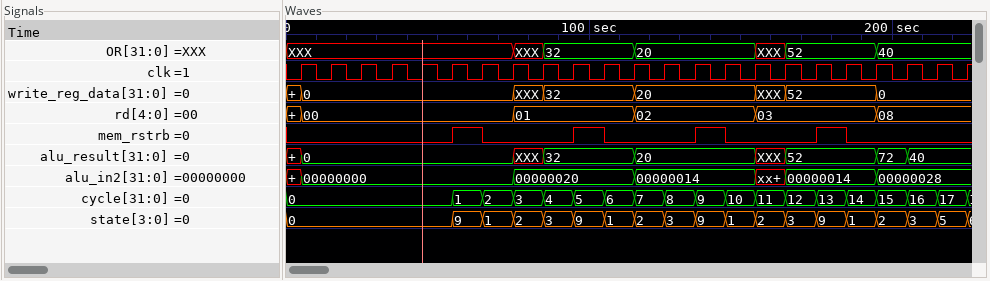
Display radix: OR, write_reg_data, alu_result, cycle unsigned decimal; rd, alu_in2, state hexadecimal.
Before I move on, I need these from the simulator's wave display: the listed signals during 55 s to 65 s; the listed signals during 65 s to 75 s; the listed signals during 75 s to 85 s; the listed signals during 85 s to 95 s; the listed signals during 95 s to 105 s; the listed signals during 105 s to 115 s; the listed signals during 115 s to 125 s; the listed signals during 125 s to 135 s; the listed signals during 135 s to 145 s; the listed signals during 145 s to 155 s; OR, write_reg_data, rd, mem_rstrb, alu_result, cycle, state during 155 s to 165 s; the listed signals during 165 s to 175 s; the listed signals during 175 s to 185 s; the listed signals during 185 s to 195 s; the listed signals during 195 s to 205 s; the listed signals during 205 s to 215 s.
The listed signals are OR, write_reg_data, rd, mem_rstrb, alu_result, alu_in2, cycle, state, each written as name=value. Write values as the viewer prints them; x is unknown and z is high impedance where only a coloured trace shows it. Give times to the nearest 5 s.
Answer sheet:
OR=XXX, write_reg_data=0, rd=00, mem_rstrb=1, alu_result=0, alu_in2=00000000, cycle=1, state=9
OR=XXX, write_reg_data=0, rd=00, mem_rstrb=0, alu_result=0, alu_in2=00000000, cycle=2, state=1
OR=XXX, write_reg_data=XXX, rd=01, mem_rstrb=0, alu_result=XXX, alu_in2=00000020, cycle=3, state=2
OR=32, write_reg_data=32, rd=01, mem_rstrb=0, alu_result=32, alu_in2=00000020, cycle=4, state=3
OR=32, write_reg_data=32, rd=01, mem_rstrb=1, alu_result=32, alu_in2=00000020, cycle=5, state=9
OR=32, write_reg_data=32, rd=01, mem_rstrb=0, alu_result=32, alu_in2=00000020, cycle=6, state=1
OR=20, write_reg_data=20, rd=02, mem_rstrb=0, alu_result=20, alu_in2=00000014, cycle=7, state=2
OR=20, write_reg_data=20, rd=02, mem_rstrb=0, alu_result=20, alu_in2=00000014, cycle=8, state=3
OR=20, write_reg_data=20, rd=02, mem_rstrb=1, alu_result=20, alu_in2=00000014, cycle=9, state=9
OR=20, write_reg_data=20, rd=02, mem_rstrb=0, alu_result=20, alu_in2=00000014, cycle=10, state=1
OR=XXX, write_reg_data=XXX, rd=03, mem_rstrb=0, alu_result=XXX, cycle=11, state=2
OR=52, write_reg_data=52, rd=03, mem_rstrb=0, alu_result=52, alu_in2=00000014, cycle=12, state=3
OR=52, write_reg_data=52, rd=03, mem_rstrb=1, alu_result=52, alu_in2=00000014, cycle=13, state=9
OR=52, write_reg_data=52, rd=03, mem_rstrb=0, alu_result=52, alu_in2=00000014, cycle=14, state=1
OR=40, write_reg_data=0, rd=08, mem_rstrb=0, alu_result=72, alu_in2=00000028, cycle=15, state=2
OR=40, write_reg_data=0, rd=08, mem_rstrb=0, alu_result=40, alu_in2=00000028, cycle=16, state=3
